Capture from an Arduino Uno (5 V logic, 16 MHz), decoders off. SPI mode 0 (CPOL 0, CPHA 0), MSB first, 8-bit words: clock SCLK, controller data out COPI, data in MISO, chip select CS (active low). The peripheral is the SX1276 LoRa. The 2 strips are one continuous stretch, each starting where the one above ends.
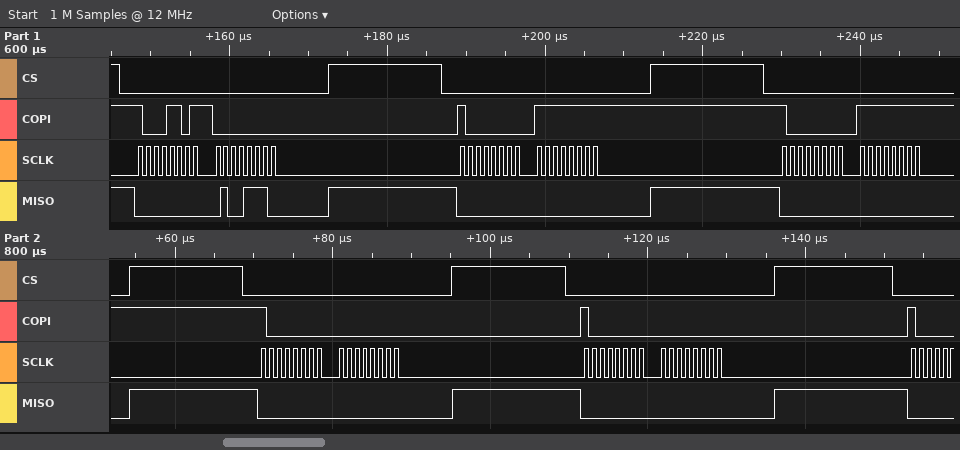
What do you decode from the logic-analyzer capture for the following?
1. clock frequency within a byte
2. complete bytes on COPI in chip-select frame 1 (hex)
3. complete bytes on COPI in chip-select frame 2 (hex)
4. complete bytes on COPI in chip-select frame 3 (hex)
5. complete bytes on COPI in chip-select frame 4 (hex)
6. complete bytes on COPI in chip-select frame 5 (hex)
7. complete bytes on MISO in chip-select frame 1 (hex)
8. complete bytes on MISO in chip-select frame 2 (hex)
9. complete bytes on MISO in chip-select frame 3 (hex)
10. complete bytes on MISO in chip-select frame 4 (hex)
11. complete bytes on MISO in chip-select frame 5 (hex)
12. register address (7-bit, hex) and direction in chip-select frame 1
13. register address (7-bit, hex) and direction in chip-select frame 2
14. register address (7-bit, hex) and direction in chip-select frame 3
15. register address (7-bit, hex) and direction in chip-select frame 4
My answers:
1 MHz
0x8D 0x00
0x80 0xFF
0x80 0xFF
0x80 0x00
0x80 0x00
0x00 0x4E
0x00 0x00
0x00 0x00
0x00 0x00
0x00 0x00
0x0D write
0x00 write
0x00 write
0x00 write
